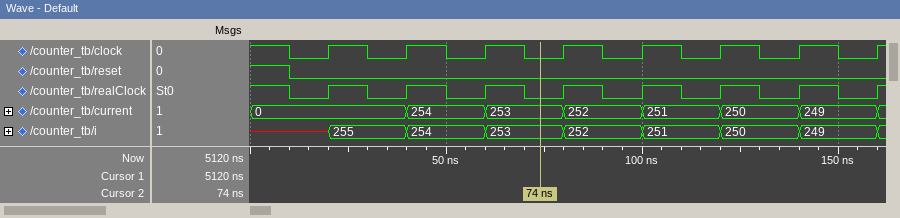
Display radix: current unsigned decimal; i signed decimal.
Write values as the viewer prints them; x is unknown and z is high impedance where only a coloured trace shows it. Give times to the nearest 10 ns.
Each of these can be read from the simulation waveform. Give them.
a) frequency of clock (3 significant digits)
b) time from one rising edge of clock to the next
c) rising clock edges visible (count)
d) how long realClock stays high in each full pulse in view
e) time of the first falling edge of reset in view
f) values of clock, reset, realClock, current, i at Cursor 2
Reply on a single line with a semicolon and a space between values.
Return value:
50.0 MHz; 20 ns; 8; 10 ns, 10 ns, 10 ns, 10 ns, 10 ns, 10 ns, 10 ns; 10 ns; clock=0, reset=0, realClock=0, current=253, i=253
